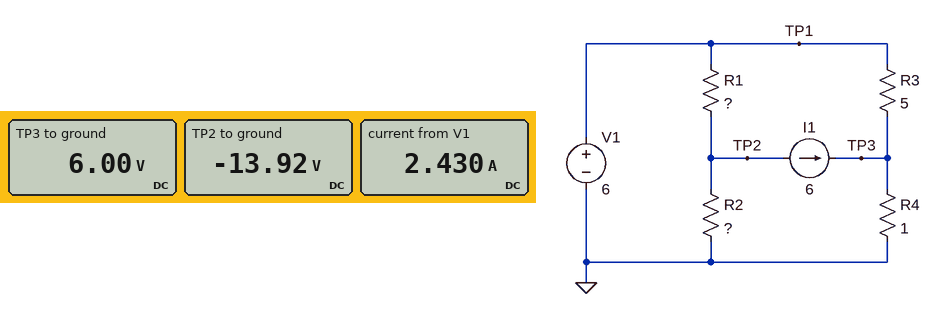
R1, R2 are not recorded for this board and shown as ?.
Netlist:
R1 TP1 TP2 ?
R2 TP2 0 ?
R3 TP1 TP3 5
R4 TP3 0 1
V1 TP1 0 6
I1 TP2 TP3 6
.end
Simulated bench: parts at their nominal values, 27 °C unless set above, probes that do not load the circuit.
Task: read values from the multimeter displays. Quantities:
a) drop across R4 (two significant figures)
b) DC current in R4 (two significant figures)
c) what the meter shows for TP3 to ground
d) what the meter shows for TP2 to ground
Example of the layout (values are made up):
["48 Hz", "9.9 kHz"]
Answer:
["6.0 V", "6.0 A", "6.00 V", "-13.92 V"]
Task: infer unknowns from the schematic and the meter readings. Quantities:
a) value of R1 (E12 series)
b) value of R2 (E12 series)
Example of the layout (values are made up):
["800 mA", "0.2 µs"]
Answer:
["8.2 Ω", "3.9 Ω"]
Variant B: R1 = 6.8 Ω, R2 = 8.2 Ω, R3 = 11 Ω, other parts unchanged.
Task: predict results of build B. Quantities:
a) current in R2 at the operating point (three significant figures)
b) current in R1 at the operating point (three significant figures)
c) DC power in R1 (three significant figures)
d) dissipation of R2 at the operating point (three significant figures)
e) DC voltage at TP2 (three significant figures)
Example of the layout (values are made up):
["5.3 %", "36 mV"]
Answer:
["2.32 A", "3.68 A", "92.1 W", "44.1 W", "-19.0 V"]
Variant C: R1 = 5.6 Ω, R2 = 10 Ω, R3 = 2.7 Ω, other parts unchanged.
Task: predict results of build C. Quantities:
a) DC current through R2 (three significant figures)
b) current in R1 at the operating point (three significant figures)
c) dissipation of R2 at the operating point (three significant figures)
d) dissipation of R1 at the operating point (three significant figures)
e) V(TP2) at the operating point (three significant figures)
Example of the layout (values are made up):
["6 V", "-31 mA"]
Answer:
["1.77 A", "4.23 A", "31.3 W", "100 W", "-17.7 V"]
